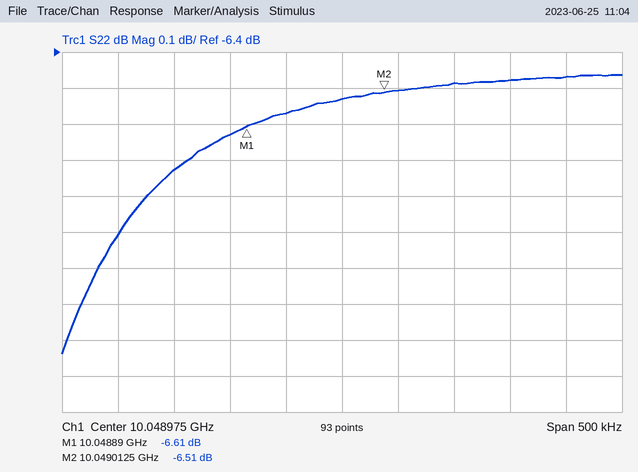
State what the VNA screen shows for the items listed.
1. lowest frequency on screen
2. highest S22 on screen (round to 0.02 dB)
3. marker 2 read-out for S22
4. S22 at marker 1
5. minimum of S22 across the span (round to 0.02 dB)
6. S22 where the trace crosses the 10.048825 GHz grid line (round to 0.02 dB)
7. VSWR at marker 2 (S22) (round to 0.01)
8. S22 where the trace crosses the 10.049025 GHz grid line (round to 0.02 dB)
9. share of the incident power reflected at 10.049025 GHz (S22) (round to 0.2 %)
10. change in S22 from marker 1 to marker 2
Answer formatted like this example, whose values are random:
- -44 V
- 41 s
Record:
- 10.048725 GHz
- -6.46 dB
- -6.51 dB
- -6.61 dB
- -7.24 dB
- -6.72 dB
- 2.79
- -6.50 dB
- 22.4 %
- 0.10 dB
